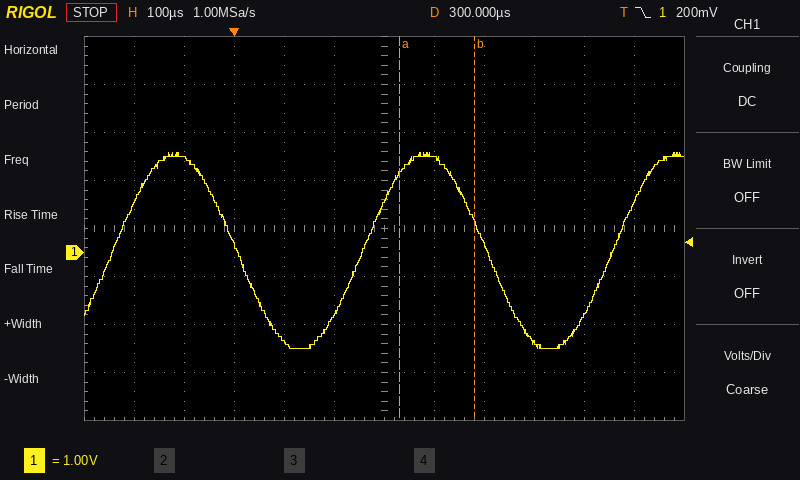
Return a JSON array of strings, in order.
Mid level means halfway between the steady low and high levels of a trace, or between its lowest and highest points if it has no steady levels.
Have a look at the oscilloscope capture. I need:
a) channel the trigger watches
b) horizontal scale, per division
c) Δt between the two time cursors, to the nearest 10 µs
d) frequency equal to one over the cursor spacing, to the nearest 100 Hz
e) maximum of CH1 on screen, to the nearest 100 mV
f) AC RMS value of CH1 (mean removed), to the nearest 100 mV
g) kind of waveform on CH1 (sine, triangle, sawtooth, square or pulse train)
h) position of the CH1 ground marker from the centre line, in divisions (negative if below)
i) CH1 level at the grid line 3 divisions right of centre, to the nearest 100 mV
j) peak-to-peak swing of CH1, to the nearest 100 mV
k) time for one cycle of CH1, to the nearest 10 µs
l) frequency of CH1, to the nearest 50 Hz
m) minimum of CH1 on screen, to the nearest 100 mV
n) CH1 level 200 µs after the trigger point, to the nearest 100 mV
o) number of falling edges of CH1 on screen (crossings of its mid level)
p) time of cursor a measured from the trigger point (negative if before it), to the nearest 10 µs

["CH1", "100 µs", "150 µs", "6.7 kHz", "2.1 V", "1.4 V", "sine", "-0.5 div", "-1.9 V", "4.1 V", "500 µs", "2.00 kHz", "-2.0 V", "-1.3 V", "2", "+330 µs"]
